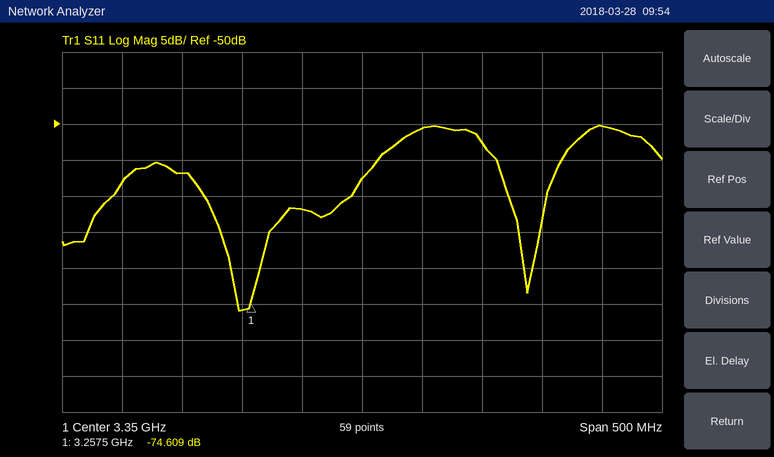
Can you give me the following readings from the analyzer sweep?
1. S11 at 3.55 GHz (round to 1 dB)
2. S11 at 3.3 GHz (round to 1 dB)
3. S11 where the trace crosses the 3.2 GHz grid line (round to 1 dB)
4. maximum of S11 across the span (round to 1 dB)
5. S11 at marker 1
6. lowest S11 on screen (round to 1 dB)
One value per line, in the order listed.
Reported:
-50 dB
-62 dB
-57 dB
-50 dB
-74.609 dB
-76 dB
